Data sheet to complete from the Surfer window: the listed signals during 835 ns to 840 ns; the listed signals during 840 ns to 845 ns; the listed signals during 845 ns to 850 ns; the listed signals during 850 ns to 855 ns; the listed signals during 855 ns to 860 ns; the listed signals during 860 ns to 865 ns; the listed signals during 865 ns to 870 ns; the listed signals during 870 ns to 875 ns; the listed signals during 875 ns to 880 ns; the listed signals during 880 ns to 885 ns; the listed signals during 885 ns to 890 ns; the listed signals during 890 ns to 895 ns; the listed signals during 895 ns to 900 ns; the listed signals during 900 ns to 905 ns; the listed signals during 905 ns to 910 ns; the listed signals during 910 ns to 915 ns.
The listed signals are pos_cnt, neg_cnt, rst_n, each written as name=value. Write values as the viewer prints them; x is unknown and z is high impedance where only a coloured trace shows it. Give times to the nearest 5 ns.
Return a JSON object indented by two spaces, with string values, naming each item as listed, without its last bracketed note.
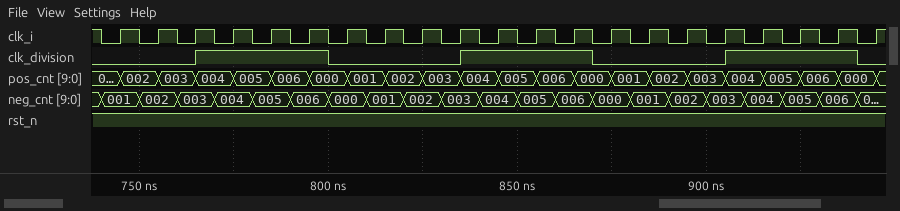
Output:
{
  "the listed signals during 835 ns to 840 ns": "pos_cnt=004, neg_cnt=003, rst_n=1",
  "the listed signals during 840 ns to 845 ns": "pos_cnt=004, neg_cnt=004, rst_n=1",
  "the listed signals during 845 ns to 850 ns": "pos_cnt=005, neg_cnt=004, rst_n=1",
  "the listed signals during 850 ns to 855 ns": "pos_cnt=005, neg_cnt=005, rst_n=1",
  "the listed signals during 855 ns to 860 ns": "pos_cnt=006, neg_cnt=005, rst_n=1",
  "the listed signals during 860 ns to 865 ns": "pos_cnt=006, neg_cnt=006, rst_n=1",
  "the listed signals during 865 ns to 870 ns": "pos_cnt=000, neg_cnt=006, rst_n=1",
  "the listed signals during 870 ns to 875 ns": "pos_cnt=000, neg_cnt=000, rst_n=1",
  "the listed signals during 875 ns to 880 ns": "pos_cnt=001, neg_cnt=000, rst_n=1",
  "the listed signals during 880 ns to 885 ns": "pos_cnt=001, neg_cnt=001, rst_n=1",
  "the listed signals during 885 ns to 890 ns": "pos_cnt=002, neg_cnt=001, rst_n=1",
  "the listed signals during 890 ns to 895 ns": "pos_cnt=002, neg_cnt=002, rst_n=1",
  "the listed signals during 895 ns to 900 ns": "pos_cnt=003, neg_cnt=002, rst_n=1",
  "the listed signals during 900 ns to 905 ns": "pos_cnt=003, neg_cnt=003, rst_n=1",
  "the listed signals during 905 ns to 910 ns": "pos_cnt=004, neg_cnt=003, rst_n=1",
  "the listed signals during 910 ns to 915 ns": "pos_cnt=004, neg_cnt=004, rst_n=1"
}
